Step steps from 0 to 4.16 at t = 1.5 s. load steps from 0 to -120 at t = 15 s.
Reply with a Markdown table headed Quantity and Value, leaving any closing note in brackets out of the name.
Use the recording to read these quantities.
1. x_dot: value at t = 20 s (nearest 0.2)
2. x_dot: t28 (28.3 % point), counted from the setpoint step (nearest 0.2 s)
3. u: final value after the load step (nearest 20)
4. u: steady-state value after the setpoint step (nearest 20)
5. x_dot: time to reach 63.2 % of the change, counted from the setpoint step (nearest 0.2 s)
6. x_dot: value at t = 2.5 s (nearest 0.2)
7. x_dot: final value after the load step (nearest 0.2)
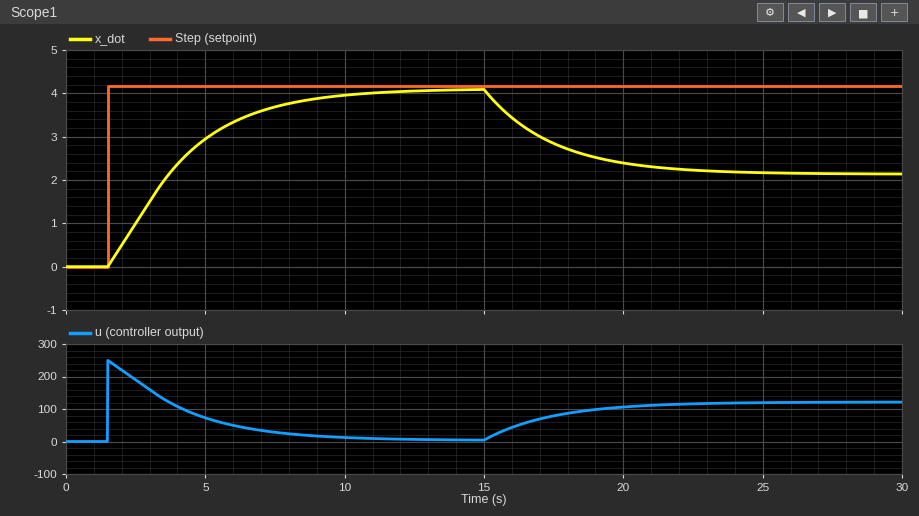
| Quantity | Value |
|---|---|
| x_dot: value at t = 20 s | 2.4 |
| x_dot: t28 (28.3 % point), counted from the setpoint step | 1.2 s |
| u: final value after the load step | 120 |
| u: steady-state value after the setpoint step | 0 |
| x_dot: time to reach 63.2 % of the change, counted from the setpoint step | 2.8 s |
| x_dot: value at t = 2.5 s | 1.0 |
| x_dot: final value after the load step | 2.2 |
